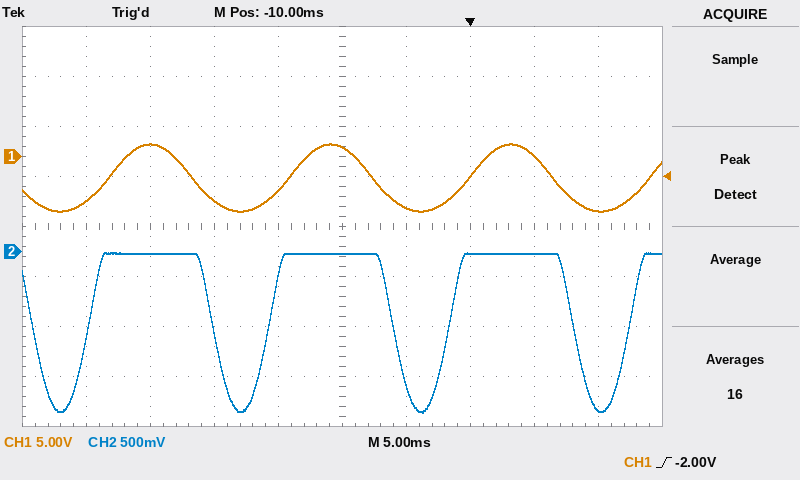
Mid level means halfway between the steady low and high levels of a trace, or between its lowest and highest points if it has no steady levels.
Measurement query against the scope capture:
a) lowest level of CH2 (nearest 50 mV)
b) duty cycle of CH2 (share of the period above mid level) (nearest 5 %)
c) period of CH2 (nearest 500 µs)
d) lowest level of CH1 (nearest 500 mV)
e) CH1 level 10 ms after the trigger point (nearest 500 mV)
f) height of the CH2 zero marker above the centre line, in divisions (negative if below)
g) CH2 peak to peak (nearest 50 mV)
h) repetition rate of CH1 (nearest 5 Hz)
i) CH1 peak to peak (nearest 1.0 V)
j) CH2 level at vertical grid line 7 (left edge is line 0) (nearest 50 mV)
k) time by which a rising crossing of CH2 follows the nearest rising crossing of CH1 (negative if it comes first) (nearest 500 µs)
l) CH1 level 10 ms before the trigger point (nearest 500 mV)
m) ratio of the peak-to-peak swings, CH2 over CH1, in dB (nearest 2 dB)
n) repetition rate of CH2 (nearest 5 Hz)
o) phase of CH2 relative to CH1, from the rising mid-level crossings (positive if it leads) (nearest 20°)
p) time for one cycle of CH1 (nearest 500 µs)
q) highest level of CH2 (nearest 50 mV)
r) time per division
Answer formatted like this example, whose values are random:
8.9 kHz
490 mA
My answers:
-1.60 V
70 %
14.0 ms
-5.5 V
-5.5 V
-0.5 div
1.60 V
70 Hz
7.0 V
0 mV
-1.5 ms
1.0 V
-12 dB
70 Hz
+40°
14.0 ms
0 mV
5 ms
